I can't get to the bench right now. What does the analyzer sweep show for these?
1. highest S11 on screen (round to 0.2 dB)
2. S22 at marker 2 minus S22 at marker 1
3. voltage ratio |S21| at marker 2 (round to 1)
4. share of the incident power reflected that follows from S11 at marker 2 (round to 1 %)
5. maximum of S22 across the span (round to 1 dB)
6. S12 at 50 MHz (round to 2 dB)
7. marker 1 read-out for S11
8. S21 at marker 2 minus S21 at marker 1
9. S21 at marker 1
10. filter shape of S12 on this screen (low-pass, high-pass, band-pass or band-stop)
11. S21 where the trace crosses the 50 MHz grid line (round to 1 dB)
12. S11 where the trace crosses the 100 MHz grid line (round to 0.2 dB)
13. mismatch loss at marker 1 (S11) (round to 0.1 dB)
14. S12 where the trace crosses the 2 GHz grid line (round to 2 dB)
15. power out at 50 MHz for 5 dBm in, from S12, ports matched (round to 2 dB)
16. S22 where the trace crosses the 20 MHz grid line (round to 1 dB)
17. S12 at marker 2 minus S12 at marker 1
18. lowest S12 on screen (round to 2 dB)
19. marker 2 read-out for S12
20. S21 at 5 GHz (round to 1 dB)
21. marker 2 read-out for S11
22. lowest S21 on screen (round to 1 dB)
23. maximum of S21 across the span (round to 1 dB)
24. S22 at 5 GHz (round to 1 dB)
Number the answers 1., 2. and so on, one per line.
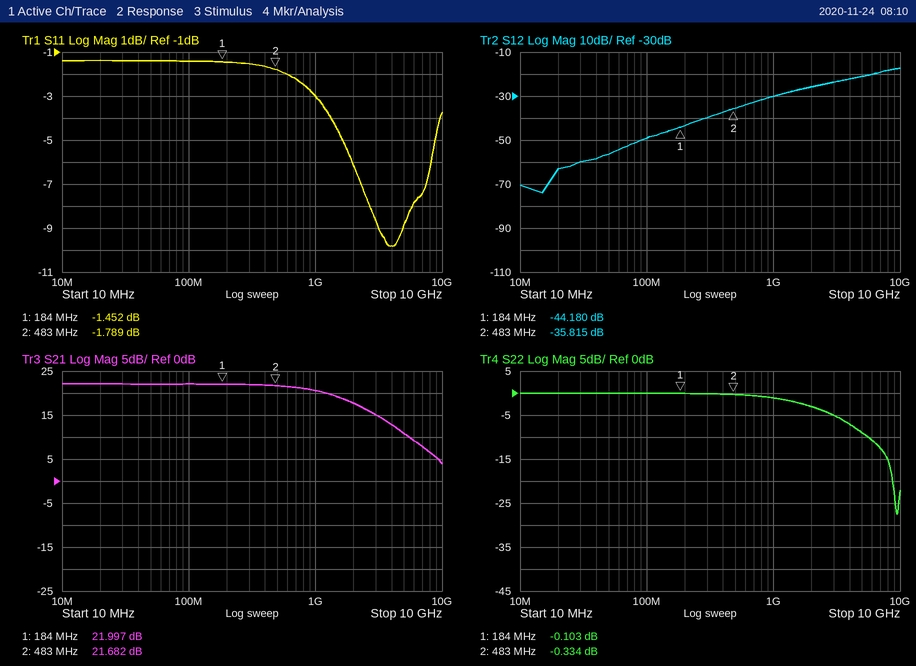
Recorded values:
1. -1.4 dB
2. -0.231 dB
3. 12
4. 66 %
5. 0 dB
6. -56 dB
7. -1.452 dB
8. -0.315 dB
9. 21.997 dB
10. high-pass
11. 22 dB
12. -1.4 dB
13. 5.5 dB
14. -26 dB
15. -52 dBm
16. 0 dB
17. 8.365 dB
18. -74 dB
19. -35.815 dB
20. 11 dB
21. -1.789 dB
22. 4 dB
23. 22 dB
24. -9 dB
